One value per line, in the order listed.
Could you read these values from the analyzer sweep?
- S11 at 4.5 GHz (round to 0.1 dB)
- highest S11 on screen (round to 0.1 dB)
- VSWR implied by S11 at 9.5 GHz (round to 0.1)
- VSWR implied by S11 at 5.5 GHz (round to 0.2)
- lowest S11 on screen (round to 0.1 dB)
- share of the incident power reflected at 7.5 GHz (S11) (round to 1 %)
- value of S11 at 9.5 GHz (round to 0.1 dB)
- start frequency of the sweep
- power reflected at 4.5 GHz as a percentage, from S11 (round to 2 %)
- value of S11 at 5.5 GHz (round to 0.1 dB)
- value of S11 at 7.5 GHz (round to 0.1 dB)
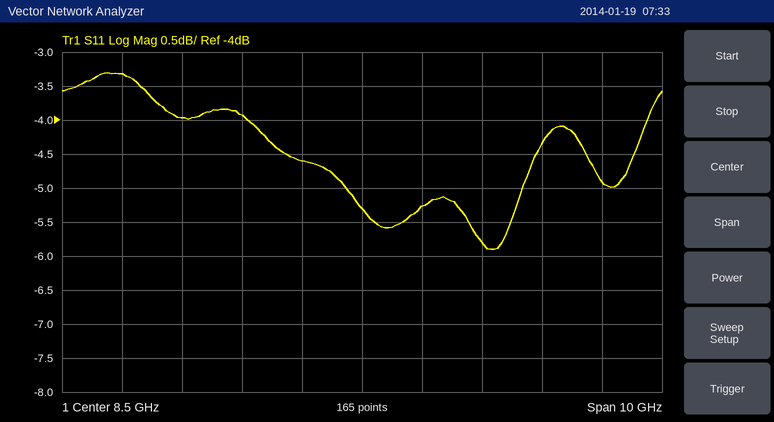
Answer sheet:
-3.3 dB
-3.3 dB
3.4
4.4
-5.9 dB
35 %
-5.3 dB
3.5 GHz
46 %
-4.0 dB
-4.6 dB
